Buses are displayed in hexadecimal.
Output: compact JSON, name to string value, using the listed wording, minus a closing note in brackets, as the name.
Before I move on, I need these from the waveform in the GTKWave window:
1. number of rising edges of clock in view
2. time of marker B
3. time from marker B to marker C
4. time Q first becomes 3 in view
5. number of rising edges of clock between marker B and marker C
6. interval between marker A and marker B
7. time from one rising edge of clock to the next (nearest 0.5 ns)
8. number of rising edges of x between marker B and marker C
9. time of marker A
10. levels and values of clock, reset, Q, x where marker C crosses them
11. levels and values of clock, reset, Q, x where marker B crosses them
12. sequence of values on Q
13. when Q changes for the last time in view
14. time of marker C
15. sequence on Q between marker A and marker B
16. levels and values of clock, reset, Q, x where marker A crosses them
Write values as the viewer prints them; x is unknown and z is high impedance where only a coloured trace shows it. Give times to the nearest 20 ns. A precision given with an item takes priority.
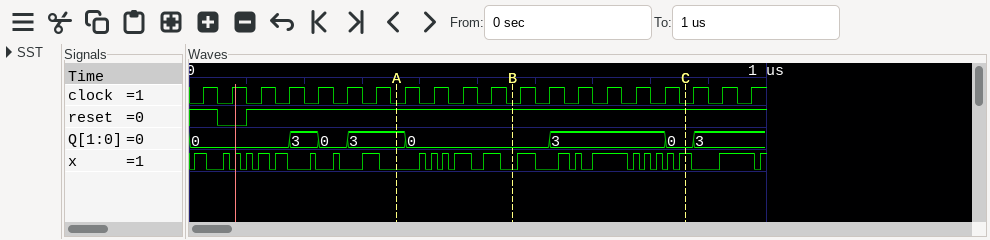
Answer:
{"number of rising edges of clock in view": "20", "time of marker B": "560 ns", "time from marker B to marker C": "300 ns", "time Q first becomes 3 in view": "180 ns", "number of rising edges of clock between marker B and marker C": "6", "interval between marker A and marker B": "200 ns", "time from one rising edge of clock to the next": "50 ns", "number of rising edges of x between marker B and marker C": "9", "time of marker A": "360 ns", "levels and values of clock, reset, Q, x where marker C crosses them": "clock=0, reset=1, Q=0, x=1", "levels and values of clock, reset, Q, x where marker B crosses them": "clock=0, reset=1, Q=0, x=0", "sequence of values on Q": "0, 3, 0, 3, 0, 3, 0, 3", "when Q changes for the last time in view": "880 ns", "time of marker C": "860 ns", "sequence on Q between marker A and marker B": "3, 0", "levels and values of clock, reset, Q, x where marker A crosses them": "clock=0, reset=1, Q=3, x=0"}
